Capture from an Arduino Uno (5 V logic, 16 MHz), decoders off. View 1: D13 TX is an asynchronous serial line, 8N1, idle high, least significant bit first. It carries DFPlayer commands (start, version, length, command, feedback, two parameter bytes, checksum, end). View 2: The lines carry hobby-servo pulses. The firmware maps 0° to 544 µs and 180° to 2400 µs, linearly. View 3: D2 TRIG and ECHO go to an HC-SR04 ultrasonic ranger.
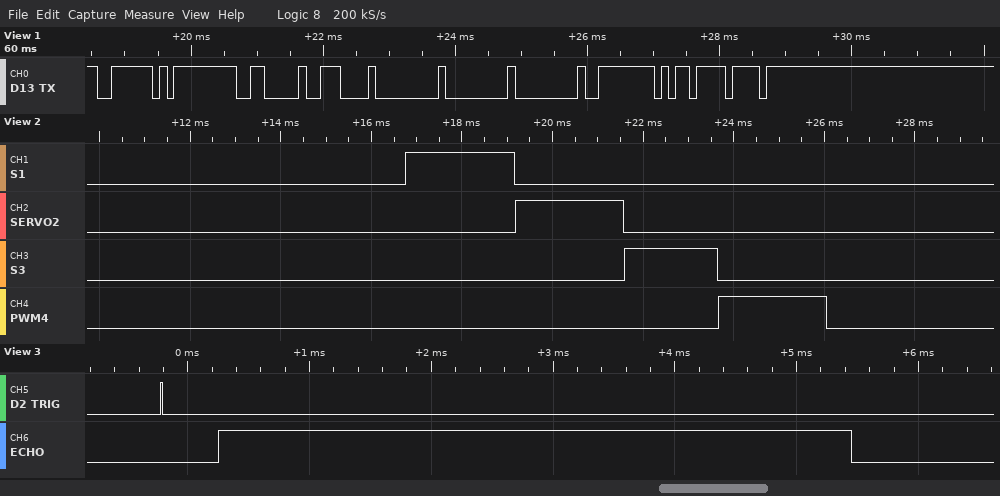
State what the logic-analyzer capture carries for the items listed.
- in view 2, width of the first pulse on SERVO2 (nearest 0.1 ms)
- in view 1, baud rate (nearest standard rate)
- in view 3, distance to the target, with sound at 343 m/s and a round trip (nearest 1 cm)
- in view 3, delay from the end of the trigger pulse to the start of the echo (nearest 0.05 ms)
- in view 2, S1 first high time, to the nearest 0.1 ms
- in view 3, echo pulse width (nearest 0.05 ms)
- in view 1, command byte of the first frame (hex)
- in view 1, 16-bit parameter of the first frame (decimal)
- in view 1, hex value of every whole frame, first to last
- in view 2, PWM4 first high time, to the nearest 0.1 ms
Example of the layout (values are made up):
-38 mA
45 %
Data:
2.4 ms
9600 baud
89 cm
0.45 ms
2.4 ms
5.20 ms
0x0E
0
7E FF 06 0E 00 00 00 FE ED EF
2.4 ms
